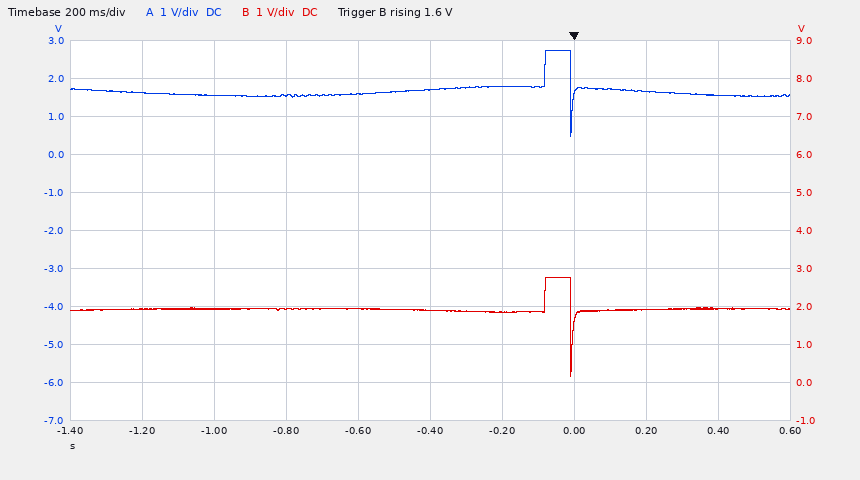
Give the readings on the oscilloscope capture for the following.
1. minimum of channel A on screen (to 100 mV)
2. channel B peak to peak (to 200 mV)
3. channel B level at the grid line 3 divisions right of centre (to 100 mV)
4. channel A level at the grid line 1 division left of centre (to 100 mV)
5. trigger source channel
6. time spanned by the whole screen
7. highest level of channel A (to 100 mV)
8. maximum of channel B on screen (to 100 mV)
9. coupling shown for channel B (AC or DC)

500 mV
2.6 V
1.9 V
1.6 V
channel B
2 s
2.7 V
2.8 V
DC
